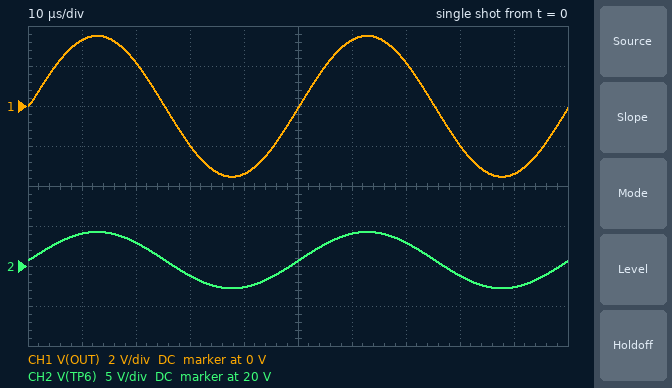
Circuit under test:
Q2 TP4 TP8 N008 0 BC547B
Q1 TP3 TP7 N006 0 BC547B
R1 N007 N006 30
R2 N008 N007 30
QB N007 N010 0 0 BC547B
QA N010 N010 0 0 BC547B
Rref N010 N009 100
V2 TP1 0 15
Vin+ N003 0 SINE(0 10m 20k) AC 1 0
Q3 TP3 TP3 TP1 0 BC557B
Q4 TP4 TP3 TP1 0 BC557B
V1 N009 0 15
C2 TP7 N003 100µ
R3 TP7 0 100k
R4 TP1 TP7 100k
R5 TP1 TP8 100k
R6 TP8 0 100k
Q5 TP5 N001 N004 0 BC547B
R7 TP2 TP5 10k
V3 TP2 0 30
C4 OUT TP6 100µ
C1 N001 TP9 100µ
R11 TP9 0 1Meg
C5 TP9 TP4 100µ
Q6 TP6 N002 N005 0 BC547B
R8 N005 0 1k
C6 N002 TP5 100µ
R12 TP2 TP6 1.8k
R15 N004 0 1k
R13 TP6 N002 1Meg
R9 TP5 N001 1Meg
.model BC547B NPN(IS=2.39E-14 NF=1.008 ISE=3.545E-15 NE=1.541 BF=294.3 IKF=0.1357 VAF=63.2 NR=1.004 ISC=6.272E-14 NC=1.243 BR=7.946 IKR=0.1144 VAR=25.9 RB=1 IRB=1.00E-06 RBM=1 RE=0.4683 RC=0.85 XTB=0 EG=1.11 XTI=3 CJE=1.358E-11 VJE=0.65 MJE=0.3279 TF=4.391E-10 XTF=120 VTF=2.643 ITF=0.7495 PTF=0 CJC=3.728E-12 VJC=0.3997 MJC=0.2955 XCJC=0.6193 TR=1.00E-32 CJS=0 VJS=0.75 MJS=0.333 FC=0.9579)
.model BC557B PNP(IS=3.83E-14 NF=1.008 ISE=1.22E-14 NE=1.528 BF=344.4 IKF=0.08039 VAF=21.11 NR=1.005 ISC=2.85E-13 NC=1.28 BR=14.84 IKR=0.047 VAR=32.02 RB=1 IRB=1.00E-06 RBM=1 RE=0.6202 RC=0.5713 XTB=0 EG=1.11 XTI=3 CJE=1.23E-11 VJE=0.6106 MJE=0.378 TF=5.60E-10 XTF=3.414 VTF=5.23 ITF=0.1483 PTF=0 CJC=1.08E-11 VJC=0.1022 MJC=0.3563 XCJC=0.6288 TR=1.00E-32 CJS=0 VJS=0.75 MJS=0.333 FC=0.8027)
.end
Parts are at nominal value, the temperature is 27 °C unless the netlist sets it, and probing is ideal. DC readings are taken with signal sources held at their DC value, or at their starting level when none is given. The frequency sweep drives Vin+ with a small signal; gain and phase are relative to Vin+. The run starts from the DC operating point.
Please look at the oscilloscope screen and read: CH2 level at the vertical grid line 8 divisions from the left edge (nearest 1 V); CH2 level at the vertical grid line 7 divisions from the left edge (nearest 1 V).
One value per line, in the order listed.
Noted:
19 V
23 V
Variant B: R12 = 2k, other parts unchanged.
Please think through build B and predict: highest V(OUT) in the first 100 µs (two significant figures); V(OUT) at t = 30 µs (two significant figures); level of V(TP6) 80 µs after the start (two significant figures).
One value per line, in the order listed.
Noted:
3.9 V
-2.2 V
18 V
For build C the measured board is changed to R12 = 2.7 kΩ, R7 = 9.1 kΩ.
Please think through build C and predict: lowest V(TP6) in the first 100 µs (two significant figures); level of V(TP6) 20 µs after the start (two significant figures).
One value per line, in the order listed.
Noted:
13 V
21 V
